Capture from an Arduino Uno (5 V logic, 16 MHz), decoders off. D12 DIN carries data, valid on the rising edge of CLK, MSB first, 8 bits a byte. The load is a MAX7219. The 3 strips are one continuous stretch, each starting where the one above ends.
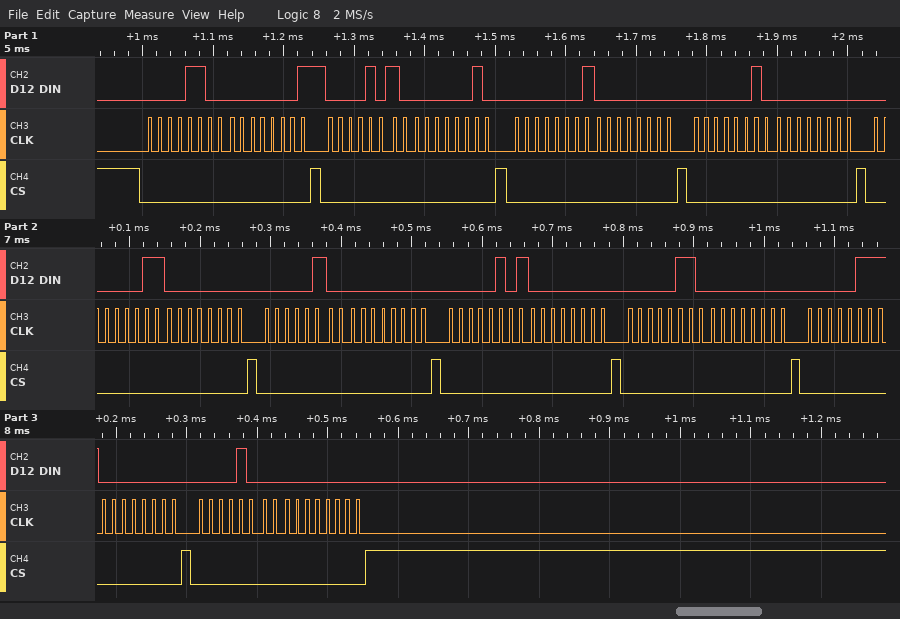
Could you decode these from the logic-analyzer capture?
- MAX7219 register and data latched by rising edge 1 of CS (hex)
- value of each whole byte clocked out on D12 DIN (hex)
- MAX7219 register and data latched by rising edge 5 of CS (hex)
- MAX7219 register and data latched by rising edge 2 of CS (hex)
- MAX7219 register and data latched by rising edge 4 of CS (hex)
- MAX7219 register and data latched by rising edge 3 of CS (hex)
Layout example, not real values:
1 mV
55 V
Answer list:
register 0xC, data 0x01
0C 01 0A 02 01 00 02 00 03 00 04 00 05 00 06 00 07 00 08 00
register 0x3, data 0x00
register 0xA, data 0x02
register 0x2, data 0x00
register 0x1, data 0x00
